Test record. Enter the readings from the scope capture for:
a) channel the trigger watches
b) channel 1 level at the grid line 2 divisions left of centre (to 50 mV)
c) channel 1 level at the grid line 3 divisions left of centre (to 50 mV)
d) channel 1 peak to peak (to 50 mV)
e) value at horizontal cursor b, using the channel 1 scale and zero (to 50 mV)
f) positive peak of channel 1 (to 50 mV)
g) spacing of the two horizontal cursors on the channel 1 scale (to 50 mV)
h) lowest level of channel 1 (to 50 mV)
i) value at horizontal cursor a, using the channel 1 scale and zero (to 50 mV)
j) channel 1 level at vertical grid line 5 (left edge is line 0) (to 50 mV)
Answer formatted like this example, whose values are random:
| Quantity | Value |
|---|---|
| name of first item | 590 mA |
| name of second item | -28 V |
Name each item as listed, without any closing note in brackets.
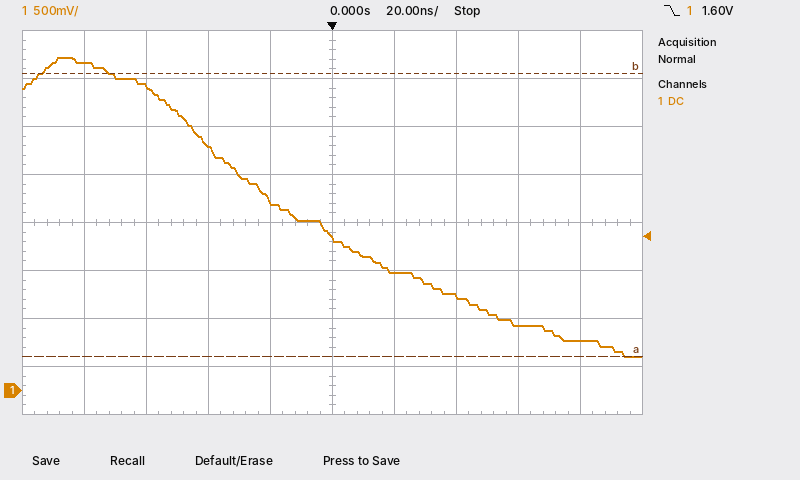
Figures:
| Quantity | Value |
|---|---|
| channel the trigger watches | channel 1 |
| channel 1 level at the grid line 2 divisions left of centre | 2.55 V |
| channel 1 level at the grid line 3 divisions left of centre | 3.15 V |
| channel 1 peak to peak | 3.10 V |
| value at horizontal cursor b, using the channel 1 scale and zero | 3.30 V |
| positive peak of channel 1 | 3.45 V |
| spacing of the two horizontal cursors on the channel 1 scale | 2.95 V |
| lowest level of channel 1 | 350 mV |
| value at horizontal cursor a, using the channel 1 scale and zero | 350 mV |
| channel 1 level at vertical grid line 5 (left edge is line 0) | 1.60 V |
